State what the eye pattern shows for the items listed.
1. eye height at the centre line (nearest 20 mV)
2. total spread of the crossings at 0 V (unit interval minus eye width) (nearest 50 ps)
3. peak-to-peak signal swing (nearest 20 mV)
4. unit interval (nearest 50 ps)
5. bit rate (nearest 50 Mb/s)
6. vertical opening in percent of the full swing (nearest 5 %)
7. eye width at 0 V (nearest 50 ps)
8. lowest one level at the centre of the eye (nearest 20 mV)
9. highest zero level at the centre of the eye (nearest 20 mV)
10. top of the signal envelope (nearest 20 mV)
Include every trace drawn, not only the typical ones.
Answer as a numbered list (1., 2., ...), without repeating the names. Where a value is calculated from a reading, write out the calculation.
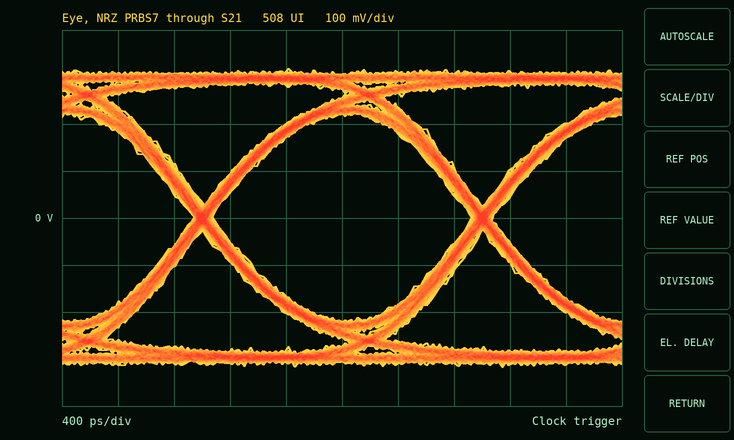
1. 440 mV
2. 150 ps
3. 640 mV
4. 2.00 ns
5. 500 Mb/s
6. 440 mV / 640 mV ≈ 68.8 %, so 70 % to the nearest 5 %
7. 1.85 ns
8. 220 mV
9. -220 mV
10. 320 mV
